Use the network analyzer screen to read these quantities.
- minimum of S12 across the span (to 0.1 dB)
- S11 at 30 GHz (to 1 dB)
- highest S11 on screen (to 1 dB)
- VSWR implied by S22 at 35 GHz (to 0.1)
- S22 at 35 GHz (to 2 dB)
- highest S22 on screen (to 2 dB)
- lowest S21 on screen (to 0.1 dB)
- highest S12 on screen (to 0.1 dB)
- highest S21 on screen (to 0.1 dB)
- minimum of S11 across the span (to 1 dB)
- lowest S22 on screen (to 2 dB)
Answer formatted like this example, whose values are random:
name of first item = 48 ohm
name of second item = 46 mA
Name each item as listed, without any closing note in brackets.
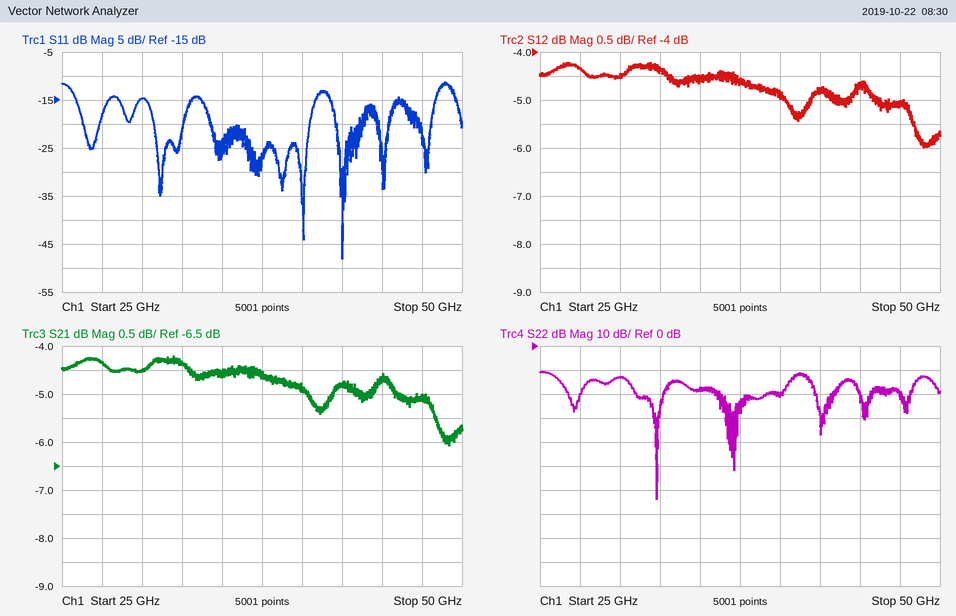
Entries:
minimum of S12 across the span = -6.0 dB
S11 at 30 GHz = -15 dB
highest S11 on screen = -11 dB
VSWR implied by S22 at 35 GHz = 1.3
S22 at 35 GHz = -18 dB
highest S22 on screen = -10 dB
lowest S21 on screen = -6.1 dB
highest S12 on screen = -4.2 dB
highest S21 on screen = -4.2 dB
minimum of S11 across the span = -48 dB
lowest S22 on screen = -64 dB
